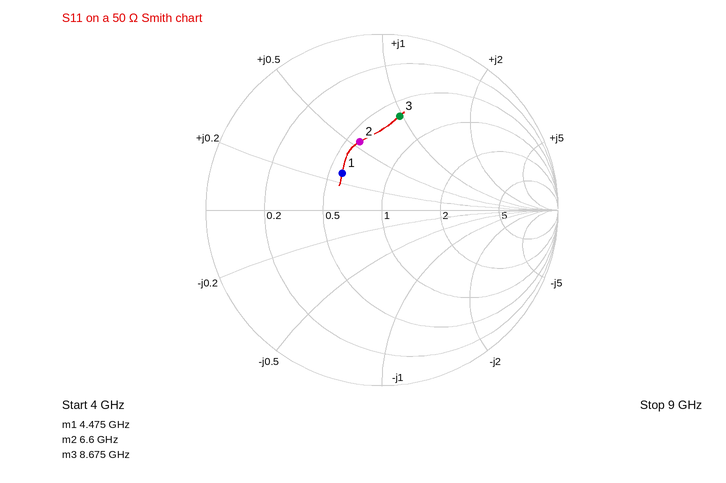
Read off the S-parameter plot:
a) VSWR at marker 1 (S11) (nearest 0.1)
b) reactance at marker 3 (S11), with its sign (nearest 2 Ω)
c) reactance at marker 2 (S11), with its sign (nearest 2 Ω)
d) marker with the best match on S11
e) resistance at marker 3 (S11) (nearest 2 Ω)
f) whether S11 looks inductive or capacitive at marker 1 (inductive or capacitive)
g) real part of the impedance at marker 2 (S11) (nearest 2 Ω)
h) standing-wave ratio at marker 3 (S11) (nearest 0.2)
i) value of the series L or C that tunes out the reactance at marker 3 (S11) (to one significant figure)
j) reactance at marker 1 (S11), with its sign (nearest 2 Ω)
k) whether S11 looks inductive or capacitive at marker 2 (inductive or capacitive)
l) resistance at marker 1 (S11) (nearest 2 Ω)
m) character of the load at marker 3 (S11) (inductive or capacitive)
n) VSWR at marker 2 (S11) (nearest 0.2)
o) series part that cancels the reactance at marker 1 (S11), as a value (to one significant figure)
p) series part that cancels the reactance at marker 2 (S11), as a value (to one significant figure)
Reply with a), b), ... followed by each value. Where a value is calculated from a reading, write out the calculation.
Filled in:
a) 1.9
b) +48 Ω
c) +28 Ω
d) marker 1
e) 32 Ω
f) inductive
g) 30 Ω
h) 3.4
i) C = 1/(2π × 8.675 GHz × 48 Ω) ≈ 382 fF, so 400 fF to one significant figure
j) +14 Ω
k) inductive
l) 30 Ω
m) inductive
n) 2.4
o) C = 1/(2π × 4.475 GHz × 14 Ω) ≈ 3 pF
p) C = 1/(2π × 6.6 GHz × 28 Ω) ≈ 861 fF, so 900 fF to one significant figure
